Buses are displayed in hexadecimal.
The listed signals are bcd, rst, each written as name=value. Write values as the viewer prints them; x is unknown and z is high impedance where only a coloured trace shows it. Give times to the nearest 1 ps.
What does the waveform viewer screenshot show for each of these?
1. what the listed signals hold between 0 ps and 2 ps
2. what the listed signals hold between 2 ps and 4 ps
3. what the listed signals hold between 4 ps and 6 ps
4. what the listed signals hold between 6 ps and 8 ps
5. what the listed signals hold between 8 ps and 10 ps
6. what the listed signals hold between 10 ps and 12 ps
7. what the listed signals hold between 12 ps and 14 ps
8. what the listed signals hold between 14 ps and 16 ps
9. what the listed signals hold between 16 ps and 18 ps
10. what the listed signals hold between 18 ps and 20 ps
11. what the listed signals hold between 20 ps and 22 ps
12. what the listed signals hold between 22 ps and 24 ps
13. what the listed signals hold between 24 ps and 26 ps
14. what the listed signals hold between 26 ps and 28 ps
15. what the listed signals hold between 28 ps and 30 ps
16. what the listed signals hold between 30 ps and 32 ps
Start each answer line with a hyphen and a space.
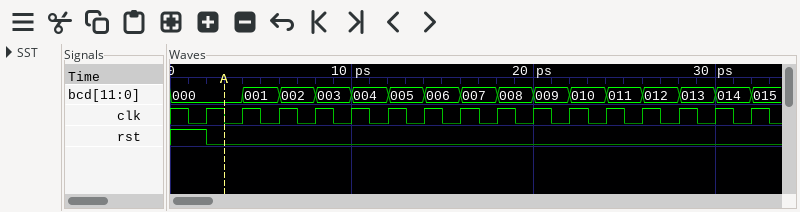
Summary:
- bcd=000, rst=1
- bcd=000, rst=0
- bcd=001, rst=0
- bcd=002, rst=0
- bcd=003, rst=0
- bcd=004, rst=0
- bcd=005, rst=0
- bcd=006, rst=0
- bcd=007, rst=0
- bcd=008, rst=0
- bcd=009, rst=0
- bcd=010, rst=0
- bcd=011, rst=0
- bcd=012, rst=0
- bcd=013, rst=0
- bcd=014, rst=0
